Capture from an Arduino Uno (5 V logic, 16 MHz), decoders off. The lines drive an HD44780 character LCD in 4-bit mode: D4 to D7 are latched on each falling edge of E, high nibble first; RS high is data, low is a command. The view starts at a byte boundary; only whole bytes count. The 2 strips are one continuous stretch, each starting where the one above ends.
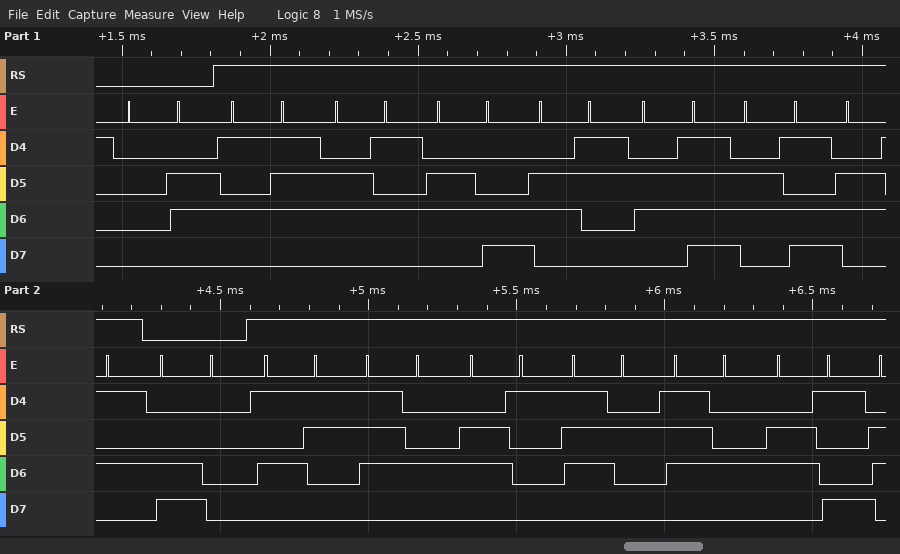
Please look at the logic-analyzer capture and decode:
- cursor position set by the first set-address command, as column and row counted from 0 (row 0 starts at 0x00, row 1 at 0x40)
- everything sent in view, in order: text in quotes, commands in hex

column 0, row 1
0x06 "Welcome" 0xC0 "Starti"
